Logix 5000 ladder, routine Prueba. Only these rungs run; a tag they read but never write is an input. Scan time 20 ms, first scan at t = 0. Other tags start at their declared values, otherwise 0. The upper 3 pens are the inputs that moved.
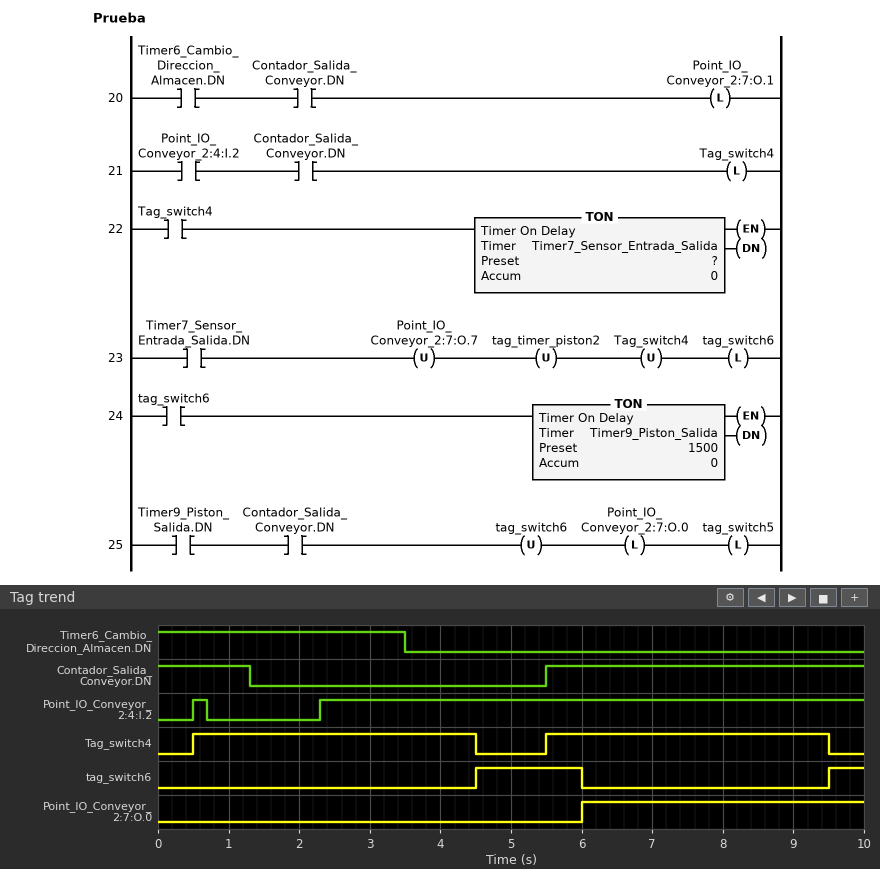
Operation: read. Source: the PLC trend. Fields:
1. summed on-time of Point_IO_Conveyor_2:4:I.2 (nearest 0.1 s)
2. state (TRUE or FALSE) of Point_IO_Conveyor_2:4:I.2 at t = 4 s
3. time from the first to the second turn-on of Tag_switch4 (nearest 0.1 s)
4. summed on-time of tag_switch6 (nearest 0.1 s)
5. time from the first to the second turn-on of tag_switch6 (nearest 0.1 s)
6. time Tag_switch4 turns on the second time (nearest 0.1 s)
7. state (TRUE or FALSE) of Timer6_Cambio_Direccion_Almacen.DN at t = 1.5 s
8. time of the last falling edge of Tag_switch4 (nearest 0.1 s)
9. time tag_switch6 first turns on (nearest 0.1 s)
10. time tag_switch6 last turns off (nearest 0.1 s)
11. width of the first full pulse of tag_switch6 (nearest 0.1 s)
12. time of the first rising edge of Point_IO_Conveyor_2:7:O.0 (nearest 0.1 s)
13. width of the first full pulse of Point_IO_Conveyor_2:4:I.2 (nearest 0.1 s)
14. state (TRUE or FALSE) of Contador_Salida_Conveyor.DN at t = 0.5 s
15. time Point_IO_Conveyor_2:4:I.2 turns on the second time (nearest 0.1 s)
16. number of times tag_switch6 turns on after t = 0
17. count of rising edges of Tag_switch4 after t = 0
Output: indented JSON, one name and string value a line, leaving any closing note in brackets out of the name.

{
  "summed on-time of Point_IO_Conveyor_2:4:I.2": "7.9 s",
  "state (TRUE or FALSE) of Point_IO_Conveyor_2:4:I.2 at t = 4 s": "TRUE",
  "time from the first to the second turn-on of Tag_switch4": "5.0 s",
  "summed on-time of tag_switch6": "2.0 s",
  "time from the first to the second turn-on of tag_switch6": "5.0 s",
  "time Tag_switch4 turns on the second time": "5.5 s",
  "state (TRUE or FALSE) of Timer6_Cambio_Direccion_Almacen.DN at t = 1.5 s": "TRUE",
  "time of the last falling edge of Tag_switch4": "9.5 s",
  "time tag_switch6 first turns on": "4.5 s",
  "time tag_switch6 last turns off": "6.0 s",
  "width of the first full pulse of tag_switch6": "1.5 s",
  "time of the first rising edge of Point_IO_Conveyor_2:7:O.0": "6.0 s",
  "width of the first full pulse of Point_IO_Conveyor_2:4:I.2": "0.2 s",
  "state (TRUE or FALSE) of Contador_Salida_Conveyor.DN at t = 0.5 s": "TRUE",
  "time Point_IO_Conveyor_2:4:I.2 turns on the second time": "2.3 s",
  "number of times tag_switch6 turns on after t = 0": "2",
  "count of rising edges of Tag_switch4 after t = 0": "2"
}
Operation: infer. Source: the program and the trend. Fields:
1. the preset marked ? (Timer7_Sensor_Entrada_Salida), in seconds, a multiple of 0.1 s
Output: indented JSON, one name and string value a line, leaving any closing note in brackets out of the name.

{
  "the preset marked ? (Timer7_Sensor_Entrada_Salida), in seconds, a multiple of 0.1 s": "4.0 s"
}
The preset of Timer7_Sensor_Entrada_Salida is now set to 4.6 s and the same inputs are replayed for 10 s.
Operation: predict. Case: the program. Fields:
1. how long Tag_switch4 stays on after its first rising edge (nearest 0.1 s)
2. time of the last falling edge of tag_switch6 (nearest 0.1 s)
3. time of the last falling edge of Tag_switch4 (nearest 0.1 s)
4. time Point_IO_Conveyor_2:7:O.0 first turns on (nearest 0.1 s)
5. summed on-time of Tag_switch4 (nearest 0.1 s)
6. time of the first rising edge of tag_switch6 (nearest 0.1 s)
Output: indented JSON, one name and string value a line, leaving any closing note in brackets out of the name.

{
  "how long Tag_switch4 stays on after its first rising edge": "4.6 s",
  "time of the last falling edge of tag_switch6": "6.6 s",
  "time of the last falling edge of Tag_switch4": "5.1 s",
  "time Point_IO_Conveyor_2:7:O.0 first turns on": "6.6 s",
  "summed on-time of Tag_switch4": "9.1 s",
  "time of the first rising edge of tag_switch6": "5.1 s"
}
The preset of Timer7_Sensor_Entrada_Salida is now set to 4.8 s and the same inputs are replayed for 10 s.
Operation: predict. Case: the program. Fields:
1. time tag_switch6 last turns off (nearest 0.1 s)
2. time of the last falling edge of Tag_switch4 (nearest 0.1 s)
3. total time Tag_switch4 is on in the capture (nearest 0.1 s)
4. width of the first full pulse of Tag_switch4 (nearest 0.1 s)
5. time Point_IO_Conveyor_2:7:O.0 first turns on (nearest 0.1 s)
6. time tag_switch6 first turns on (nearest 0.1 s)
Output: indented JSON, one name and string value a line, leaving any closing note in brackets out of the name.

{
  "time tag_switch6 last turns off": "6.8 s",
  "time of the last falling edge of Tag_switch4": "5.3 s",
  "total time Tag_switch4 is on in the capture": "9.3 s",
  "width of the first full pulse of Tag_switch4": "4.8 s",
  "time Point_IO_Conveyor_2:7:O.0 first turns on": "6.8 s",
  "time tag_switch6 first turns on": "5.3 s"
}
